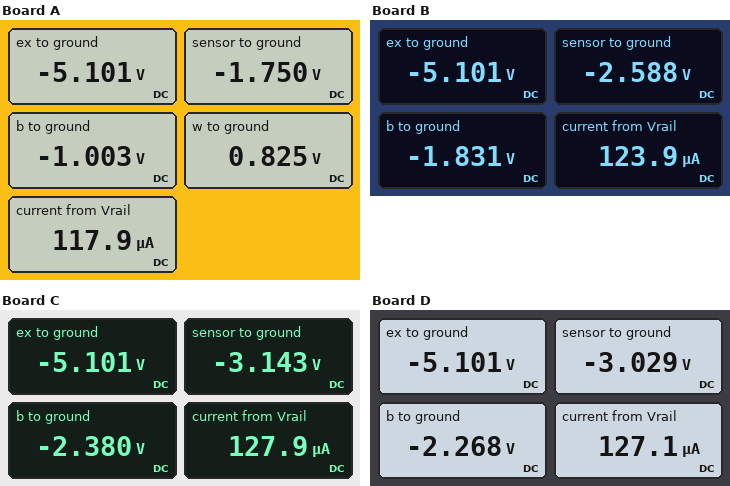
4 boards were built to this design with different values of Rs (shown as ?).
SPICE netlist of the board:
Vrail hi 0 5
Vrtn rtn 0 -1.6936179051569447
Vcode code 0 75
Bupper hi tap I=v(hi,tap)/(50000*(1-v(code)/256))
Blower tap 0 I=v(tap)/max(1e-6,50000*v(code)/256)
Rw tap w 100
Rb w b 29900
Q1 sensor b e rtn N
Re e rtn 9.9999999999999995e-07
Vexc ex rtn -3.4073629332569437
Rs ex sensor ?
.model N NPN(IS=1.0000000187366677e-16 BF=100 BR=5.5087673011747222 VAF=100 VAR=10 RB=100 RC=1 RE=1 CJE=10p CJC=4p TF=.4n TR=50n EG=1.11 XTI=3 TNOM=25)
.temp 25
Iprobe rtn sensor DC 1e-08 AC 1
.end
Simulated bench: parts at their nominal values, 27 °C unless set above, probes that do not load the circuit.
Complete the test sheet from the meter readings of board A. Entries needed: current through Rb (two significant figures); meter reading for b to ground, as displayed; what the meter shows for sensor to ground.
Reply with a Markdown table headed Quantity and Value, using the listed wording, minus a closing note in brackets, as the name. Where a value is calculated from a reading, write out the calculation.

| Quantity | Value |
|---|---|
| current through Rb | (825 mV - (-1.003 V)) / 29.9 kΩ = 61 µA |
| meter reading for b to ground, as displayed | -1.003 V |
| what the meter shows for sensor to ground | -1.750 V |
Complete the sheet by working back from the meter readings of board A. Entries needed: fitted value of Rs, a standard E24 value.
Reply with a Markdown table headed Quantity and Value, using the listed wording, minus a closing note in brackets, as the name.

| Quantity | Value |
|---|---|
| fitted value of Rs, a standard E24 value | 10 kΩ |
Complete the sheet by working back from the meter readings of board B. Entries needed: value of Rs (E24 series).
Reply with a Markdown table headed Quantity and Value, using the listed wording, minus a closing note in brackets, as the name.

| Quantity | Value |
|---|---|
| value of Rs | 4.7 kΩ |
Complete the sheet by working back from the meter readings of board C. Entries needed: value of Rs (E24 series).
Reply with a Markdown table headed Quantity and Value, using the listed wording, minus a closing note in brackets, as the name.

| Quantity | Value |
|---|---|
| value of Rs | 3 kΩ |
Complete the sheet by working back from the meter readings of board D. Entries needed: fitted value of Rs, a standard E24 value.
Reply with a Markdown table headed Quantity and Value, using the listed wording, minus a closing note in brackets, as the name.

| Quantity | Value |
|---|---|
| fitted value of Rs, a standard E24 value | 3.3 kΩ |
